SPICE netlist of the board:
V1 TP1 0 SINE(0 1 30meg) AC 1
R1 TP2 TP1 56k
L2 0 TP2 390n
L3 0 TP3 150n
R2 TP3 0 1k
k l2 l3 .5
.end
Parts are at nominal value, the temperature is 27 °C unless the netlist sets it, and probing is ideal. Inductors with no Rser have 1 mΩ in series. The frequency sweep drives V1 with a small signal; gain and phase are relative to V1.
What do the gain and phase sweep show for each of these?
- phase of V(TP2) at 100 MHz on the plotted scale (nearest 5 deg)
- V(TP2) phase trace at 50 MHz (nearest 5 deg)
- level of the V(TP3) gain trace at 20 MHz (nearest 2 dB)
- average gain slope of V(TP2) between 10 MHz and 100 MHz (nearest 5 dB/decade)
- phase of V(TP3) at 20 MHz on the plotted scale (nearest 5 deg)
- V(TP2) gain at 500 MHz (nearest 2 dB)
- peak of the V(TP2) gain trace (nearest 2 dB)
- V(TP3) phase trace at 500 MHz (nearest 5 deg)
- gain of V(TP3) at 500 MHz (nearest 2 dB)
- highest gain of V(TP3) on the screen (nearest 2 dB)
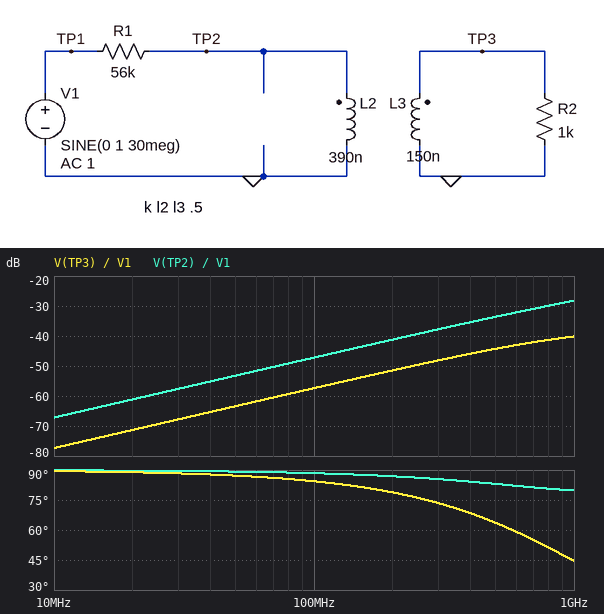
90 deg
90 deg
-72 dB
20 dB/decade
90 deg
-34 dB
-28 dB
65 deg
-44 dB
-40 dB
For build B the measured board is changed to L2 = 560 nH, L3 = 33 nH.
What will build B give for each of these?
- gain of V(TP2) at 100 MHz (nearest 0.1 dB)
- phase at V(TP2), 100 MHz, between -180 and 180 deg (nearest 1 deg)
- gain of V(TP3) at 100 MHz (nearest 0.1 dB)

-44.0 dB
89 deg
-62.4 dB
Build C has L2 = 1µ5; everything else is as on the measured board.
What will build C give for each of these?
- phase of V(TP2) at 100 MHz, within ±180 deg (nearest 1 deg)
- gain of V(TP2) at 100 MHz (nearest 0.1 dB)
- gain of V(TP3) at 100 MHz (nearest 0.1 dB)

88 deg
-35.5 dB
-51.5 dB
